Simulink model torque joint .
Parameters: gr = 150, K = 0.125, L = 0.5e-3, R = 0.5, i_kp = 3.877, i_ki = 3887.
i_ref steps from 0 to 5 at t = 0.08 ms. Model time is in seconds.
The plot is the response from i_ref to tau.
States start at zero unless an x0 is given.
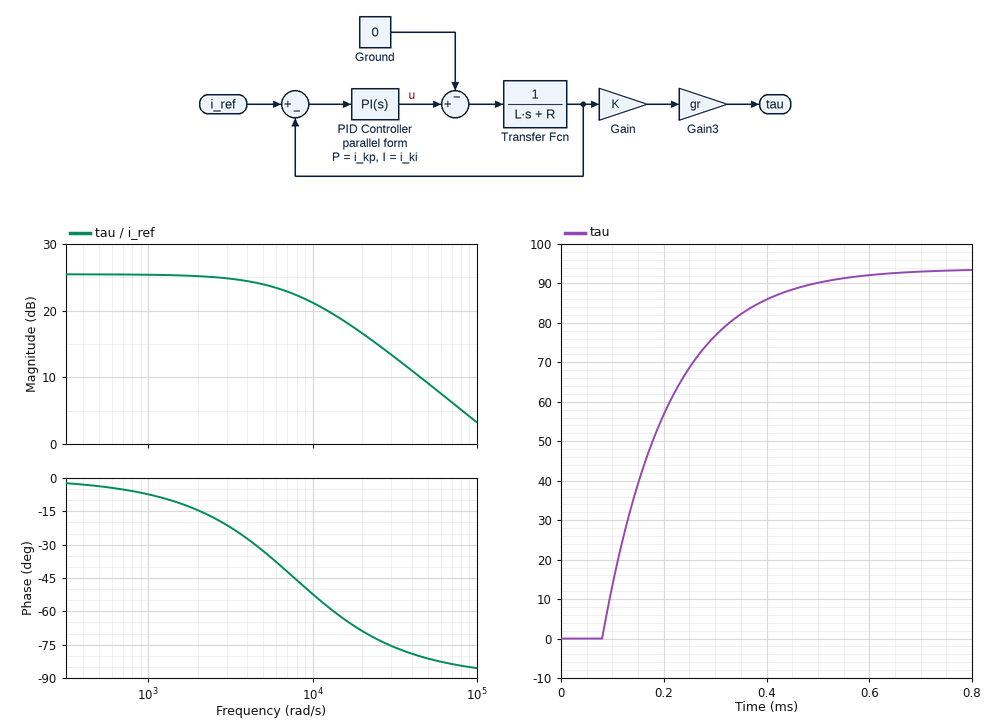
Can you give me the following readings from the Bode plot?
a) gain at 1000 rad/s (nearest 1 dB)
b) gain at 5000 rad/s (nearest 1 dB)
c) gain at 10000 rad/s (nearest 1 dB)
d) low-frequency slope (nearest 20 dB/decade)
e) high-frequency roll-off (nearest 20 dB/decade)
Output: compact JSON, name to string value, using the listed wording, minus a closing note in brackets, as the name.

{"gain at 1000 rad/s": "25 dB", "gain at 5000 rad/s": "24 dB", "gain at 10000 rad/s": "21 dB", "low-frequency slope": "0 dB/decade", "high-frequency roll-off": "-20 dB/decade"}
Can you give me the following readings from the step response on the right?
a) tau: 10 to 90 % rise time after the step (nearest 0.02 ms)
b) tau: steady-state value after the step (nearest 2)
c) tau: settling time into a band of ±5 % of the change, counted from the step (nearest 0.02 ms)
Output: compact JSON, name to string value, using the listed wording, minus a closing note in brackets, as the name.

{"tau: 10 to 90 % rise time after the step": "0.28 ms", "tau: steady-state value after the step": "94", "tau: settling time into a band of ±5 % of the change, counted from the step": "0.38 ms"}
